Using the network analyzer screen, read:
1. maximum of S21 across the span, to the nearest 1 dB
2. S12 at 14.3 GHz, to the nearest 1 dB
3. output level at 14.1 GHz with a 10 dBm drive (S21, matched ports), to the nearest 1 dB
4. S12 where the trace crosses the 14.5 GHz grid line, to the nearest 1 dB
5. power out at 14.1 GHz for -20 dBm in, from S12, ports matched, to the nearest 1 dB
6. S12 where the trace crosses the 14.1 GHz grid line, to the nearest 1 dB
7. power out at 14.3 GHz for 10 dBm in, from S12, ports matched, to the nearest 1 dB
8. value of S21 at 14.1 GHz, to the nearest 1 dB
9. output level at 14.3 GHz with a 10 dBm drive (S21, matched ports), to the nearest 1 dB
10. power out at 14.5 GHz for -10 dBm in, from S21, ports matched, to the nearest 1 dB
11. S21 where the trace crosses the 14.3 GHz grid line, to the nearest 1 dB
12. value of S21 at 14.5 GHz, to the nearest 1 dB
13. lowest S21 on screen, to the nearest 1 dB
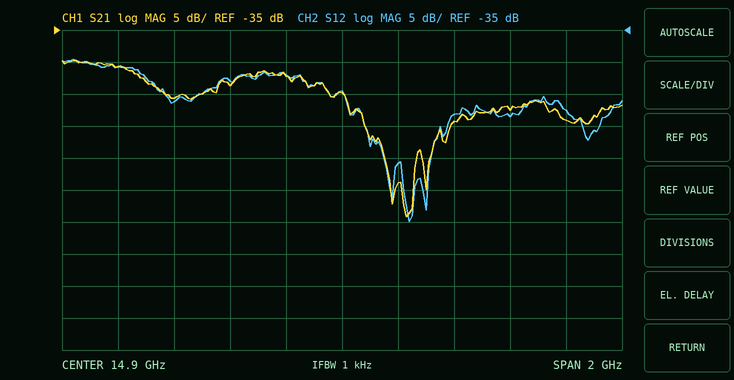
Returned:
-40 dB
-46 dB
-31 dBm
-43 dB
-61 dBm
-41 dB
-36 dBm
-41 dB
-36 dBm
-54 dBm
-46 dB
-44 dB
-64 dB
